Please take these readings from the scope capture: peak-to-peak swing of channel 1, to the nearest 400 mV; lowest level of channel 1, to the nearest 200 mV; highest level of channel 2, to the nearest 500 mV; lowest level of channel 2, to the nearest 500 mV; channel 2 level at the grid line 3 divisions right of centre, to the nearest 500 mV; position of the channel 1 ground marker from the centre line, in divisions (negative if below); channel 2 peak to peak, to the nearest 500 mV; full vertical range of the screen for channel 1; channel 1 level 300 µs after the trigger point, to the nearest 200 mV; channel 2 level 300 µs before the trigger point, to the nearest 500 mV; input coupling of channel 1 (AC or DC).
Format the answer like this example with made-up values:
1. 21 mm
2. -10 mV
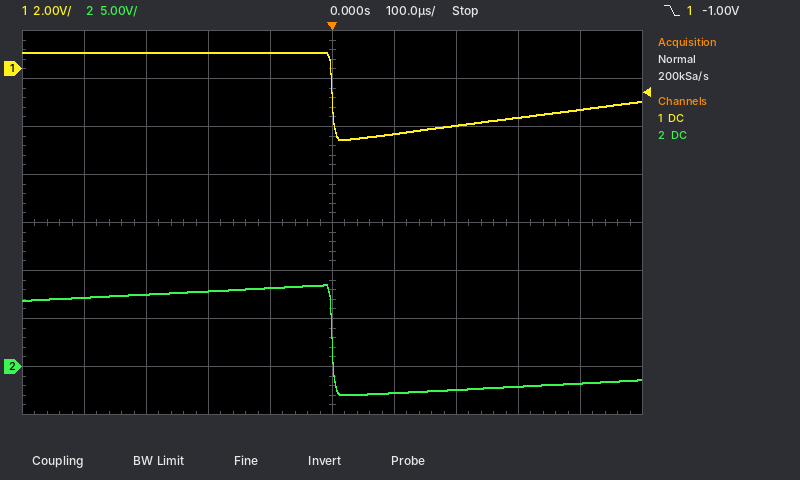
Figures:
1. 3.6 V
2. -3.0 V
3. 8.5 V
4. -3.0 V
5. -2.0 V
6. +3.2 div
7. 11.5 V
8. 16 V
9. -2.0 V
10. 7.5 V
11. DC
